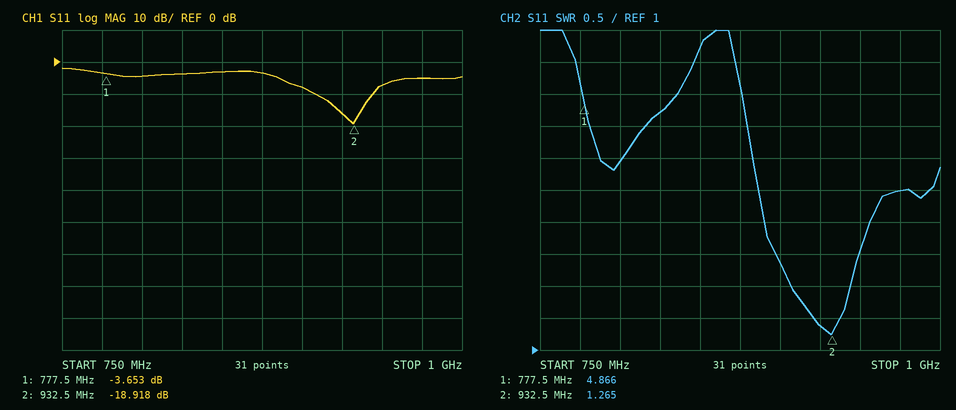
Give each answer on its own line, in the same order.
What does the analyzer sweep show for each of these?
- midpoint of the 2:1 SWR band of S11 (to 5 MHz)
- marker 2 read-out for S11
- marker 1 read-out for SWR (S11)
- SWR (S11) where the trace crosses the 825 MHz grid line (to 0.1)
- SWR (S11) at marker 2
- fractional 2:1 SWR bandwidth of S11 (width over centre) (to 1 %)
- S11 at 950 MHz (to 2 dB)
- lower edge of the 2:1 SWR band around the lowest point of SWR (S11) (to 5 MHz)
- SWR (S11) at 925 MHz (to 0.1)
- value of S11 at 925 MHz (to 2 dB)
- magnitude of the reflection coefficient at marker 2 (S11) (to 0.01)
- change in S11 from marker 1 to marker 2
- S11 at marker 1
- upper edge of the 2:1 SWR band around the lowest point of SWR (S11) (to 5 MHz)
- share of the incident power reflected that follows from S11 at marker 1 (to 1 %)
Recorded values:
925 MHz
-18.918 dB
4.866
4.7
1.265
4 %
-8 dB
905 MHz
1.4
-16 dB
0.11
-15.265 dB
-3.653 dB
945 MHz
43 %
